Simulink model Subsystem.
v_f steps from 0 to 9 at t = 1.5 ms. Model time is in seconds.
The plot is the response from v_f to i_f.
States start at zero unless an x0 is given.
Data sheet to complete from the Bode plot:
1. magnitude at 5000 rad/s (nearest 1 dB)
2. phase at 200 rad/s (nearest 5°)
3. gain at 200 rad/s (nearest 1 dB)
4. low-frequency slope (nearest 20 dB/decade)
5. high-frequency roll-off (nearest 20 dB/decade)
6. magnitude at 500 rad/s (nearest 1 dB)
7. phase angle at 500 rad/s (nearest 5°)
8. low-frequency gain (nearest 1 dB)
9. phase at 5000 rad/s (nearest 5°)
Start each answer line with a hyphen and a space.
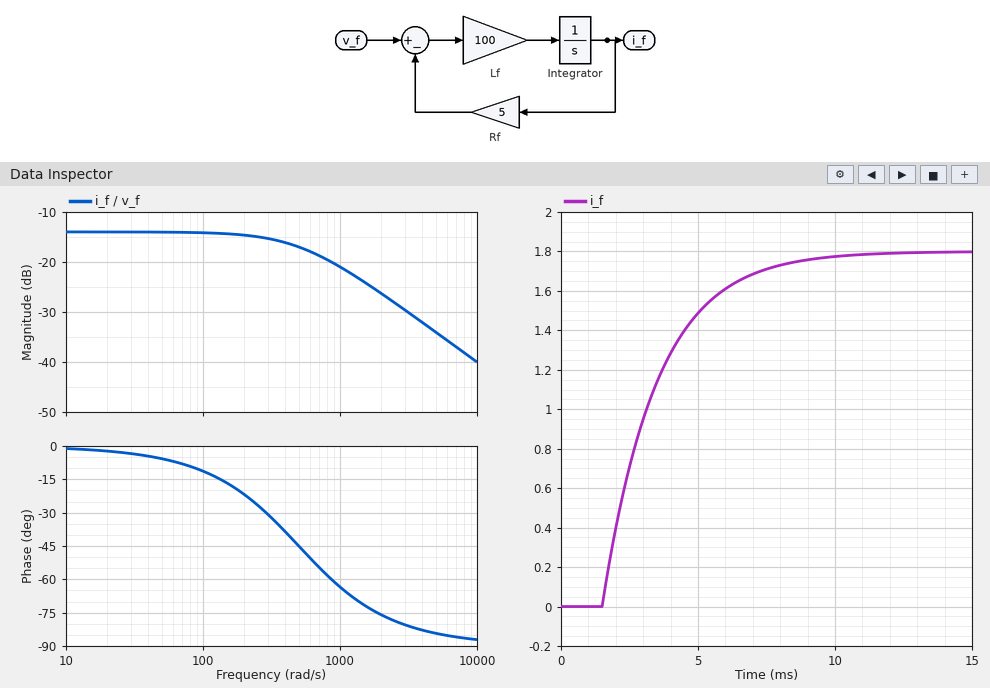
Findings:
- -34 dB
- -20°
- -15 dB
- 0 dB/decade
- -20 dB/decade
- -17 dB
- -45°
- -14 dB
- -85°
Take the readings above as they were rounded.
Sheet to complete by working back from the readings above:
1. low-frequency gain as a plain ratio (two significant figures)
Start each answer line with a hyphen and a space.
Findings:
- 0.20
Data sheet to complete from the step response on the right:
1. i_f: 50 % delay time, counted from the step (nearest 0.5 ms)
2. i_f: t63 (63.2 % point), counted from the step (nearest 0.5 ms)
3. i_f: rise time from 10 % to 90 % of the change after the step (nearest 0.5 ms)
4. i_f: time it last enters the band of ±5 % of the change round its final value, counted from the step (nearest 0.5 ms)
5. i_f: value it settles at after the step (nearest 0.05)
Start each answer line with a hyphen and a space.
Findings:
- 1.5 ms
- 2.0 ms
- 4.5 ms
- 6.0 ms
- 1.80
